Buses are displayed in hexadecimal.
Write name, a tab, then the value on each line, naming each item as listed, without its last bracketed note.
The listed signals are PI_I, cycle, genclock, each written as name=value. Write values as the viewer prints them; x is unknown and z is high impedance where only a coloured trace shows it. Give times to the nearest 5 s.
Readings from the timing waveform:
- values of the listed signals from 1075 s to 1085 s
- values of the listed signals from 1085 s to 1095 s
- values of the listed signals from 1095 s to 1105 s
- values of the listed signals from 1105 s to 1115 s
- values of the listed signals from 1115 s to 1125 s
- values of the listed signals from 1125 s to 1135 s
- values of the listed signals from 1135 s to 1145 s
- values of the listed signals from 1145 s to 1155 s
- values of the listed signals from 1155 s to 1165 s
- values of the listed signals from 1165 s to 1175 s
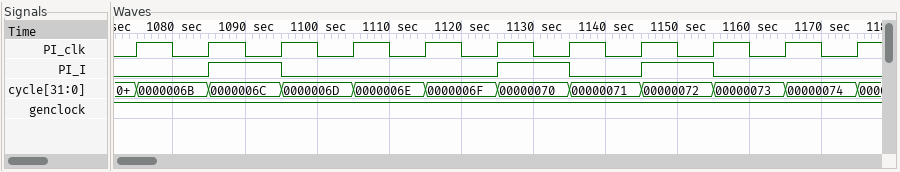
values of the listed signals from 1075 s to 1085 s	PI_I=0, cycle=0000006B, genclock=1
values of the listed signals from 1085 s to 1095 s	PI_I=1, cycle=0000006C, genclock=1
values of the listed signals from 1095 s to 1105 s	PI_I=0, cycle=0000006D, genclock=1
values of the listed signals from 1105 s to 1115 s	PI_I=0, cycle=0000006E, genclock=1
values of the listed signals from 1115 s to 1125 s	PI_I=0, cycle=0000006F, genclock=1
values of the listed signals from 1125 s to 1135 s	PI_I=1, cycle=00000070, genclock=1
values of the listed signals from 1135 s to 1145 s	PI_I=0, cycle=00000071, genclock=1
values of the listed signals from 1145 s to 1155 s	PI_I=1, cycle=00000072, genclock=1
values of the listed signals from 1155 s to 1165 s	PI_I=0, cycle=00000073, genclock=1
values of the listed signals from 1165 s to 1175 s	PI_I=0, cycle=00000074, genclock=1
